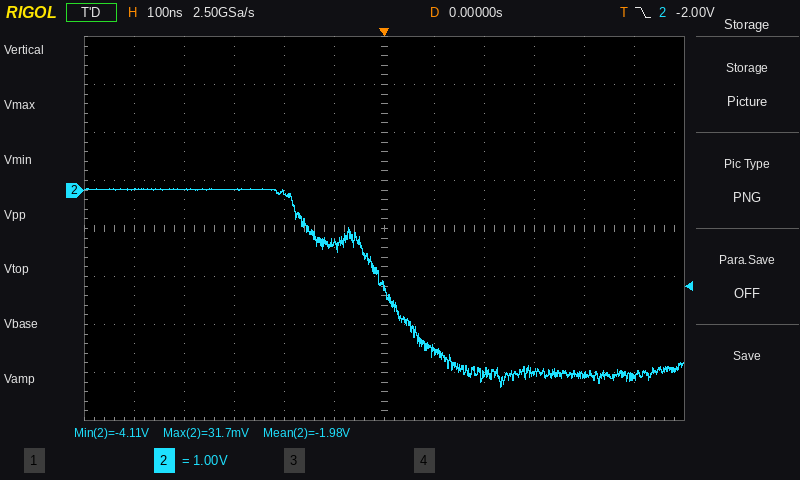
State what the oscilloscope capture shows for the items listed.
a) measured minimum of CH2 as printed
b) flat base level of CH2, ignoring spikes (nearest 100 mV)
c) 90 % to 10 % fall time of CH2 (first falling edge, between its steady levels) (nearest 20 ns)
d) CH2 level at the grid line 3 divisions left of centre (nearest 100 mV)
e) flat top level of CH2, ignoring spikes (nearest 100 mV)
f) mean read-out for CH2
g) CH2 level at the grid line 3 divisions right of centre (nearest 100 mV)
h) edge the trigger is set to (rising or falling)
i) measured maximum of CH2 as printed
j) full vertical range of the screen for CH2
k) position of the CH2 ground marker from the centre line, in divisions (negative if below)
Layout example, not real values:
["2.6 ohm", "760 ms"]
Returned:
["-4.11 V", "-3.8 V", "300 ns", "0.0 V", "0.0 V", "-1.98 V", "-3.8 V", "falling", "31.7 mV", "8 V", "+0.8 div"]
